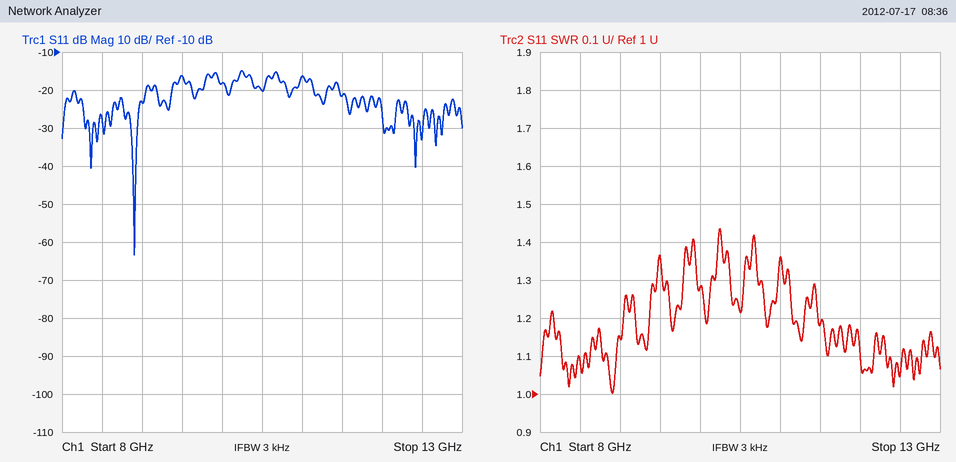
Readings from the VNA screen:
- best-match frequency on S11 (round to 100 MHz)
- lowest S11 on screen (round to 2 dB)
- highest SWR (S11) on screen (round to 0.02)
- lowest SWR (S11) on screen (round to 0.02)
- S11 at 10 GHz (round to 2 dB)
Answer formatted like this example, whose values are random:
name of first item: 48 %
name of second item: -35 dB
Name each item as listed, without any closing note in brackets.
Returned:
best-match frequency on S11: 8.9 GHz
lowest S11 on screen: -64 dB
highest SWR (S11) on screen: 1.44
lowest SWR (S11) on screen: 1.00
S11 at 10 GHz: -18 dB
